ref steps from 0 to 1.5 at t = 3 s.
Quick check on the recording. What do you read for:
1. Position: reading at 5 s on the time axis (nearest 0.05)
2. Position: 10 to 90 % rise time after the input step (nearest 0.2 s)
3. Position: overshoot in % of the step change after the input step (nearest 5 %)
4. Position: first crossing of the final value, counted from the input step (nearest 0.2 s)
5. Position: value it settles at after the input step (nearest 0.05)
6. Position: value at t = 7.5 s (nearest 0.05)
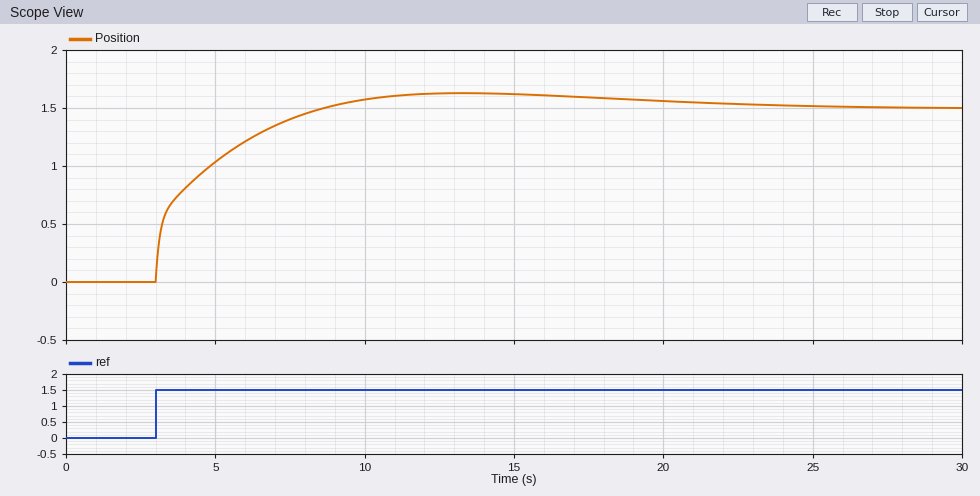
1.05
4.0 s
10 %
5.6 s
1.50
1.40
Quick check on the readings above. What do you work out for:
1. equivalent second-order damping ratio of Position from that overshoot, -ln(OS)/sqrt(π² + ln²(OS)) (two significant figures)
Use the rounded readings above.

0.59
